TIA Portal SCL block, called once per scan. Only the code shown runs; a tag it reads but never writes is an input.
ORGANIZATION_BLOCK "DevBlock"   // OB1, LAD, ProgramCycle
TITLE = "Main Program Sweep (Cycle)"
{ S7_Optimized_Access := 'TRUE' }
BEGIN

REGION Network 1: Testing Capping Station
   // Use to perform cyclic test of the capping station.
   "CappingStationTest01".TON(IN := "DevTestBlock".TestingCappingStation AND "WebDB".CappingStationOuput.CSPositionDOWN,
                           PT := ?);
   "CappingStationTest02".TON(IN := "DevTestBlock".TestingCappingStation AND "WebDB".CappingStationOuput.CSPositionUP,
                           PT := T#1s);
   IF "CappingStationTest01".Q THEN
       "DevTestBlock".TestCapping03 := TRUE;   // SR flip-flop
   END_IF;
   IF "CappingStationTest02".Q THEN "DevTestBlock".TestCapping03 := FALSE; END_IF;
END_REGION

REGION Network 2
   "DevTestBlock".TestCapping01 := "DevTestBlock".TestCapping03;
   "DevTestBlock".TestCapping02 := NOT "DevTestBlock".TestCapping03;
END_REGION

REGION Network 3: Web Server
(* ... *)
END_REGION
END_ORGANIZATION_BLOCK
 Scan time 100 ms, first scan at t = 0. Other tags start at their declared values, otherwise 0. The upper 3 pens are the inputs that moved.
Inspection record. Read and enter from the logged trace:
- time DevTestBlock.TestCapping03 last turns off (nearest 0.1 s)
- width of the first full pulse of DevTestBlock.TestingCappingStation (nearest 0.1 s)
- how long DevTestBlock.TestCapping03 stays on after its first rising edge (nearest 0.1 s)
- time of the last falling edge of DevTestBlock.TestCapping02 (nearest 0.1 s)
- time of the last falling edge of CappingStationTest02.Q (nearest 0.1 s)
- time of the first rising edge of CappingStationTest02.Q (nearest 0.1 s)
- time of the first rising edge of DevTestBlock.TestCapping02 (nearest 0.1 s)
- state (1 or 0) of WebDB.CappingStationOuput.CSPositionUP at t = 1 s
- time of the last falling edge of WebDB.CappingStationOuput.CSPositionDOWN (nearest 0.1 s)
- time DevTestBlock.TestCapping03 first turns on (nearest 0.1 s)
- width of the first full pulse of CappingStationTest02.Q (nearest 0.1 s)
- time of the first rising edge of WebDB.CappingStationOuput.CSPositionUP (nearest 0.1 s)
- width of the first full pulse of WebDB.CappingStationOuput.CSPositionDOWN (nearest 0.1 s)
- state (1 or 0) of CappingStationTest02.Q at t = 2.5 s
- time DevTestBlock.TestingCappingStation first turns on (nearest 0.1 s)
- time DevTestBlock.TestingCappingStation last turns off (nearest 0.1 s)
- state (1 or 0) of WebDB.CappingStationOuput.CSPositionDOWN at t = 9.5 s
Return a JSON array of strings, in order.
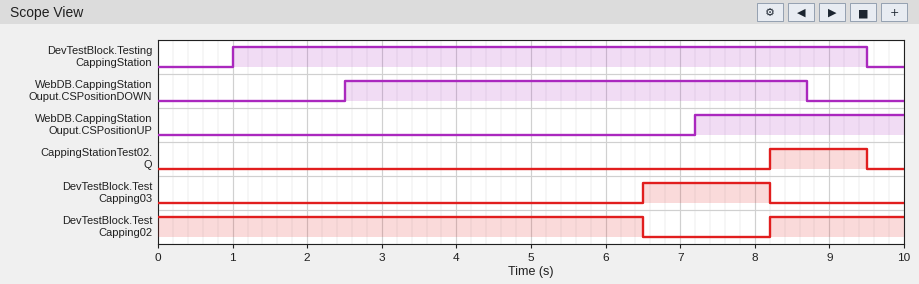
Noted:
["8.2 s", "8.5 s", "1.7 s", "6.5 s", "9.5 s", "8.2 s", "8.2 s", "0", "8.7 s", "6.5 s", "1.3 s", "7.2 s", "6.2 s", "0", "1.0 s", "9.5 s", "0"]
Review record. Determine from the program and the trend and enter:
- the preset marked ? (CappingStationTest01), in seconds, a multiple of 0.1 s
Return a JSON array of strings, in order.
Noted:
["4.0 s"]
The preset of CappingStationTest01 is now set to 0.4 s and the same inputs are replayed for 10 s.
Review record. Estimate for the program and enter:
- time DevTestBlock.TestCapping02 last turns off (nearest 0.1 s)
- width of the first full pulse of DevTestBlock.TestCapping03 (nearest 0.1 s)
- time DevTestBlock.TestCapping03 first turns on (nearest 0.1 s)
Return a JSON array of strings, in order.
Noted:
["2.9 s", "5.3 s", "2.9 s"]
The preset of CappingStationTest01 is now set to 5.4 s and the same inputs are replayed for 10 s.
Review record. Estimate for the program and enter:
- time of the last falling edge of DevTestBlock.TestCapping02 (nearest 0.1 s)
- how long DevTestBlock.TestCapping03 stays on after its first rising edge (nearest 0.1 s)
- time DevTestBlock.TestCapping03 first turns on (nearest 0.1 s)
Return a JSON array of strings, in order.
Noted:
["7.9 s", "0.3 s", "7.9 s"]
